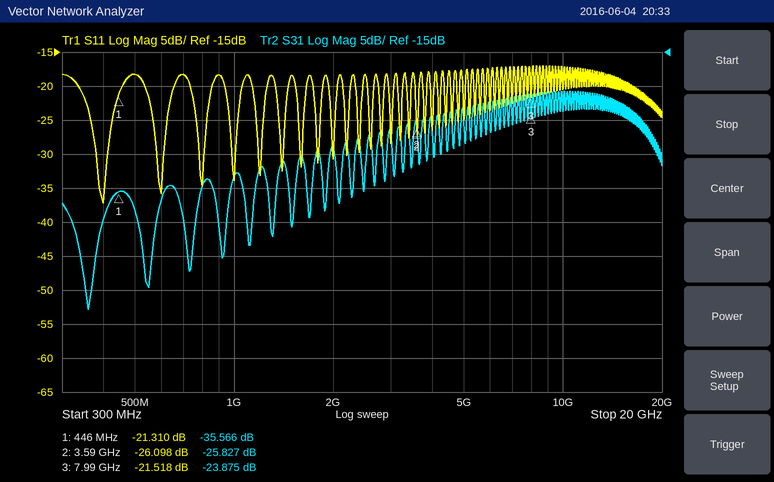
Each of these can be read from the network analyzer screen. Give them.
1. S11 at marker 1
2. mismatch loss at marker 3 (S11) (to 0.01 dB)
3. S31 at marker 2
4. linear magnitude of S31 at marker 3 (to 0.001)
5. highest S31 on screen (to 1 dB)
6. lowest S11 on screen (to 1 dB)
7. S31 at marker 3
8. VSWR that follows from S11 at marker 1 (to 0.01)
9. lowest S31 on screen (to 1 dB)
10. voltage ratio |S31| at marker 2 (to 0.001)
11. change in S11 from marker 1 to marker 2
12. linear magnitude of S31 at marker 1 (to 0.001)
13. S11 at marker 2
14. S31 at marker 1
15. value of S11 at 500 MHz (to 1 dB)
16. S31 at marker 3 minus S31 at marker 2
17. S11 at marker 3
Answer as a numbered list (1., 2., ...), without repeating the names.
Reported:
1. -21.310 dB
2. 0.03 dB
3. -25.827 dB
4. 0.064
5. -21 dB
6. -37 dB
7. -23.875 dB
8. 1.19
9. -53 dB
10. 0.051
11. -4.788 dB
12. 0.017
13. -26.098 dB
14. -35.566 dB
15. -18 dB
16. 1.952 dB
17. -21.518 dB
